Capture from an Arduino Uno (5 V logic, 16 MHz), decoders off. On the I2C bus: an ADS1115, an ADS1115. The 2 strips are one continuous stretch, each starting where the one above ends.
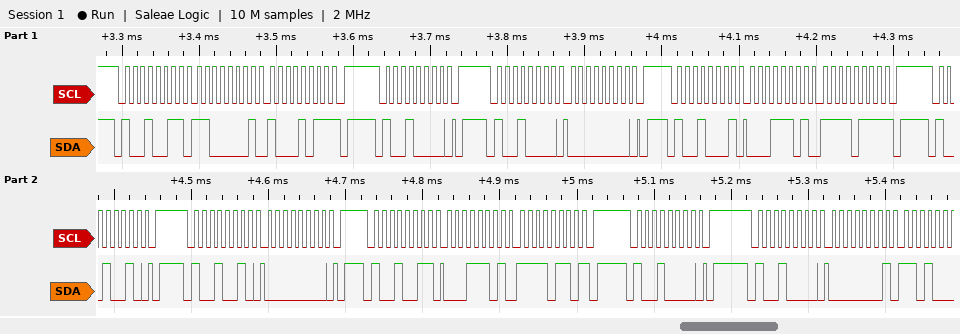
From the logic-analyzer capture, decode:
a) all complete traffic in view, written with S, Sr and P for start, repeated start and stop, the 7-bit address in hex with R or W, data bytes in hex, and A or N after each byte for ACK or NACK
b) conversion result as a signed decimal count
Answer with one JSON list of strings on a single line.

["S 49R A C1 A 8B N P S 48W A P S 48W A 00 A P S 48R A 1D A F7 N P S 49W A P S 49W A 00 A P S 49R A 1D A F6 N P S 48W A P S 48W A 01 A", "7671"]
